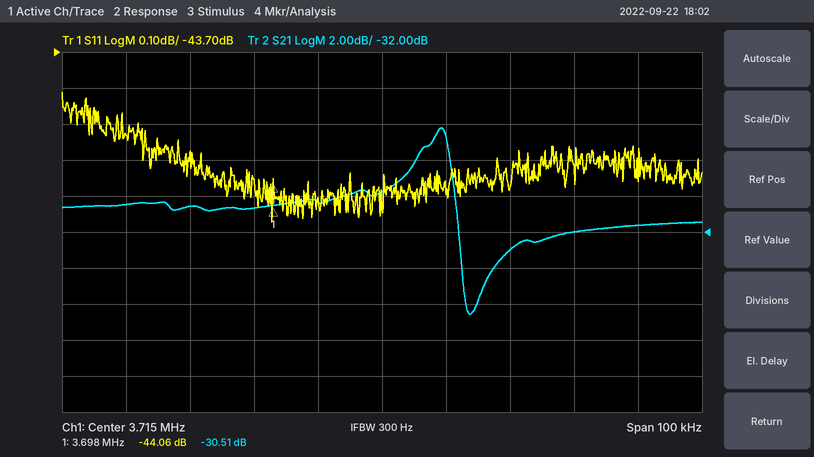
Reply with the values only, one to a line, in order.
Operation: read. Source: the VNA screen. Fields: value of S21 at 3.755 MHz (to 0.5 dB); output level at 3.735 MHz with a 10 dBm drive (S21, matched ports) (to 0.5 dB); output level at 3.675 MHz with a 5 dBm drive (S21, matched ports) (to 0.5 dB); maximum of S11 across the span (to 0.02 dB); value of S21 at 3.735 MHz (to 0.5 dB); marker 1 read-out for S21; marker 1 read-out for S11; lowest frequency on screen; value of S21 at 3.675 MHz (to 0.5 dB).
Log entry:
-31.5 dB
-23.0 dBm
-25.5 dBm
-43.82 dB
-33.0 dB
-30.51 dB
-44.06 dB
3.665 MHz
-30.5 dB
